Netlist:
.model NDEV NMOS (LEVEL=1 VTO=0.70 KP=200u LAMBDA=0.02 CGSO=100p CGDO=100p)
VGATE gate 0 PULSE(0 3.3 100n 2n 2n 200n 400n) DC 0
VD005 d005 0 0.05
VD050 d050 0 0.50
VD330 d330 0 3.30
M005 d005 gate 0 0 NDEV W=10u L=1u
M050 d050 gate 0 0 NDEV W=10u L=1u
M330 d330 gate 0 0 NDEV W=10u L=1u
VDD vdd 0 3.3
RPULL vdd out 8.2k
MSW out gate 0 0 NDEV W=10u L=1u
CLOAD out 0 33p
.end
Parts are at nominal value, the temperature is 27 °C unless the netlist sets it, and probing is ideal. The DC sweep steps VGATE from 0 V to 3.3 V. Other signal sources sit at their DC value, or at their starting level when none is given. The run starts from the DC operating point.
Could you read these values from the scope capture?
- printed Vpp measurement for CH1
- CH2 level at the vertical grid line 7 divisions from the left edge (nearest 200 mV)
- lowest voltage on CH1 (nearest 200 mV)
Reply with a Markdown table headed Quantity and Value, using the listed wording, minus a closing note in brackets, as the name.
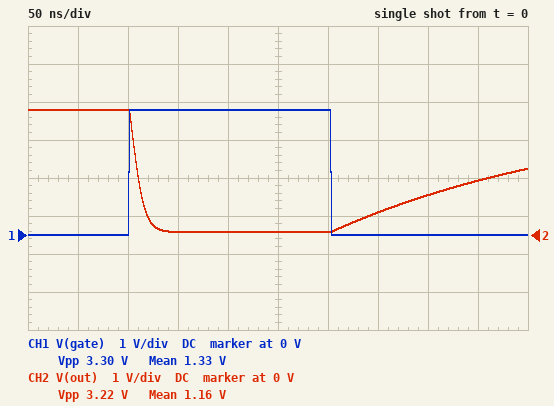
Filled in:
| Quantity | Value |
|---|---|
| printed Vpp measurement for CH1 | 3.30 V |
| CH2 level at the vertical grid line 7 divisions from the left edge | 600 mV |
| lowest voltage on CH1 | 0 V |
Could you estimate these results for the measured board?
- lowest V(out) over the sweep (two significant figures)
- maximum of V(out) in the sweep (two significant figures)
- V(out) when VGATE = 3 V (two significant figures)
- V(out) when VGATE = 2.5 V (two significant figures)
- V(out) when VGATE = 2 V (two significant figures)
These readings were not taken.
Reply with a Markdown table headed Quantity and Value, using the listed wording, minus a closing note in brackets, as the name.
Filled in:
| Quantity | Value |
|---|---|
| lowest V(out) over the sweep | 77 mV |
| maximum of V(out) in the sweep | 3.3 V |
| V(out) when VGATE = 3 V | 87 mV |
| V(out) when VGATE = 2.5 V | 110 mV |
| V(out) when VGATE = 2 V | 160 mV |
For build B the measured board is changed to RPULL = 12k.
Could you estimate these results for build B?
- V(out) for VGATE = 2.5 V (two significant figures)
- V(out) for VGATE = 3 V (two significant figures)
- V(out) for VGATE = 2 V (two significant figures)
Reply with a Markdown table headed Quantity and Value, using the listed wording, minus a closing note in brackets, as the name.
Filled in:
| Quantity | Value |
|---|---|
| V(out) for VGATE = 2.5 V | 76 mV |
| V(out) for VGATE = 3 V | 59 mV |
| V(out) for VGATE = 2 V | 110 mV |
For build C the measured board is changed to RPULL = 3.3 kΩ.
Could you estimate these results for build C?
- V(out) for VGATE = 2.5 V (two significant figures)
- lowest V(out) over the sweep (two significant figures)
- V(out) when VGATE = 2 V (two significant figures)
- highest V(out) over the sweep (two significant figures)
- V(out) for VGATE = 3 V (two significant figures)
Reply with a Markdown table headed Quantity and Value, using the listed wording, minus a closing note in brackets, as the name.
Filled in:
| Quantity | Value |
|---|---|
| V(out) for VGATE = 2.5 V | 270 mV |
| lowest V(out) over the sweep | 190 mV |
| V(out) when VGATE = 2 V | 400 mV |
| highest V(out) over the sweep | 3.3 V |
| V(out) for VGATE = 3 V | 210 mV |
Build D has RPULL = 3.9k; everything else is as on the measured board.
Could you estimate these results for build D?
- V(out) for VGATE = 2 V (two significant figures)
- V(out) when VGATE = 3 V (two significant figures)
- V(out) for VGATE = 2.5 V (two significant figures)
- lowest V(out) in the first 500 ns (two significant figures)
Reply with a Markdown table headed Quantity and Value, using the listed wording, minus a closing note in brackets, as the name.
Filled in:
| Quantity | Value |
|---|---|
| V(out) for VGATE = 2 V | 330 mV |
| V(out) when VGATE = 3 V | 180 mV |
| V(out) for VGATE = 2.5 V | 230 mV |
| lowest V(out) in the first 500 ns | 160 mV |
